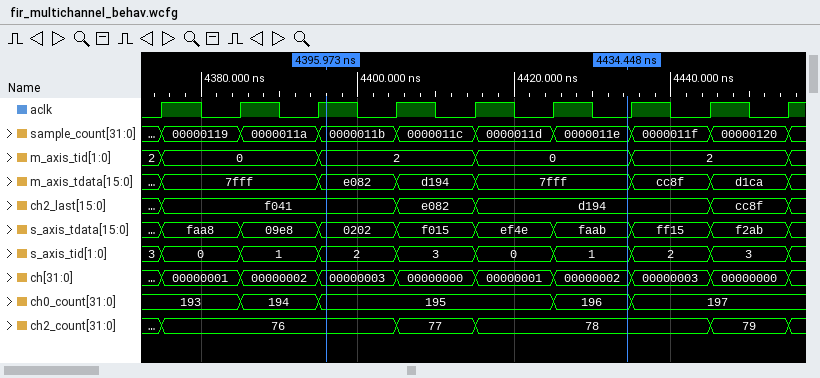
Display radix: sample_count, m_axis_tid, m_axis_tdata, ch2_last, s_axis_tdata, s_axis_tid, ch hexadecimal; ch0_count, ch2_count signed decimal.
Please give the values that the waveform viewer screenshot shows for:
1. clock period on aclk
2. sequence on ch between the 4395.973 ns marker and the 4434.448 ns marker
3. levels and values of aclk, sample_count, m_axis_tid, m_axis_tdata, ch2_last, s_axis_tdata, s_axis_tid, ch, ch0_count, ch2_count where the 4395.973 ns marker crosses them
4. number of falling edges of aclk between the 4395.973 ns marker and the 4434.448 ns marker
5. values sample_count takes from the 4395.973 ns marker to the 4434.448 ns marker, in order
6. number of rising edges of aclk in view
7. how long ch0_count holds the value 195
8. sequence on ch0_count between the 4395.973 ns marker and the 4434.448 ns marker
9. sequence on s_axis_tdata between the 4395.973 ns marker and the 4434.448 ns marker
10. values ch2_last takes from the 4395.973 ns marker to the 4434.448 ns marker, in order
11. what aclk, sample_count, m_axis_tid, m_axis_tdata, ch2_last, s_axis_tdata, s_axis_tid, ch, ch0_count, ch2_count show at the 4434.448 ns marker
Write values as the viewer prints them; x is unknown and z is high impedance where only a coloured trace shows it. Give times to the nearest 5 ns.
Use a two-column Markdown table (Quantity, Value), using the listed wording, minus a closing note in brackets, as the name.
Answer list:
| Quantity | Value |
|---|---|
| clock period on aclk | 10 ns |
| sequence on ch between the 4395.973 ns marker and the 4434.448 ns marker | 00000003, 00000000, 00000001, 00000002 |
| levels and values of aclk, sample_count, m_axis_tid, m_axis_tdata, ch2_last, s_axis_tdata, s_axis_tid, ch, ch0_count, ch2_count where the 4395.973 ns marker crosses them | aclk=1, sample_count=0000011b, m_axis_tid=2, m_axis_tdata=e082, ch2_last=f041, s_axis_tdata=0202, s_axis_tid=2, ch=00000003, ch0_count=195, ch2_count=76 |
| number of falling edges of aclk between the 4395.973 ns marker and the 4434.448 ns marker | 4 |
| values sample_count takes from the 4395.973 ns marker to the 4434.448 ns marker, in order | 0000011b, 0000011c, 0000011d, 0000011e |
| number of rising edges of aclk in view | 9 |
| how long ch0_count holds the value 195 | 30 ns |
| sequence on ch0_count between the 4395.973 ns marker and the 4434.448 ns marker | 195, 196 |
| sequence on s_axis_tdata between the 4395.973 ns marker and the 4434.448 ns marker | 0202, f015, ef4e, faab |
| values ch2_last takes from the 4395.973 ns marker to the 4434.448 ns marker, in order | f041, e082, d194 |
| what aclk, sample_count, m_axis_tid, m_axis_tdata, ch2_last, s_axis_tdata, s_axis_tid, ch, ch0_count, ch2_count show at the 4434.448 ns marker | aclk=0, sample_count=0000011e, m_axis_tid=0, m_axis_tdata=7fff, ch2_last=d194, s_axis_tdata=faab, s_axis_tid=1, ch=00000002, ch0_count=196, ch2_count=78 |
